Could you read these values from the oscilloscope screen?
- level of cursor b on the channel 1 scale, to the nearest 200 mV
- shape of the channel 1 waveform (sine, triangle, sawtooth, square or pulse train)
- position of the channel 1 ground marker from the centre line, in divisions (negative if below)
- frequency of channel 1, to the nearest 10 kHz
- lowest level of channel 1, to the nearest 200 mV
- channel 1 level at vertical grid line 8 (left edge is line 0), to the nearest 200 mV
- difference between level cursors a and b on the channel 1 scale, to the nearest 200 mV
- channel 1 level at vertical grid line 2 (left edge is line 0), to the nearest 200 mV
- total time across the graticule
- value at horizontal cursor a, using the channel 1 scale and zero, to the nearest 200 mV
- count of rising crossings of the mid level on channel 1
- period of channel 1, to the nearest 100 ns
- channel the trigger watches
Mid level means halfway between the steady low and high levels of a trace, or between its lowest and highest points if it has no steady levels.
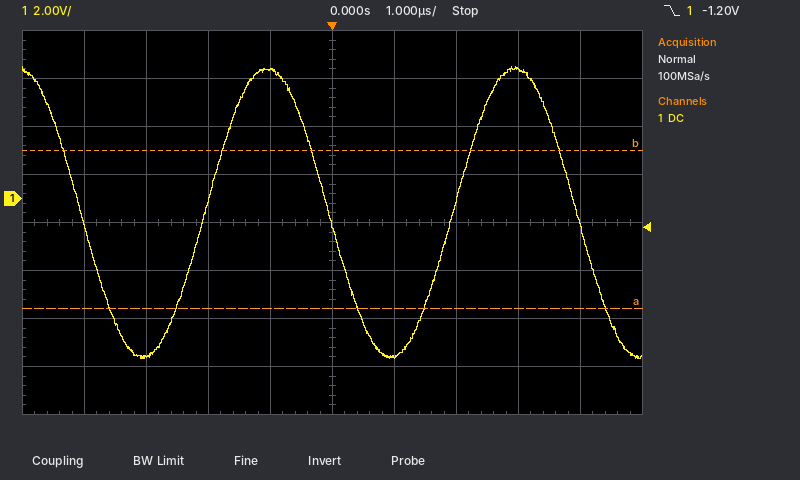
2.0 V
sine
+0.5 div
250 kHz
-6.6 V
5.4 V
6.6 V
-6.6 V
10 µs
-4.6 V
2
4.0 µs
channel 1
